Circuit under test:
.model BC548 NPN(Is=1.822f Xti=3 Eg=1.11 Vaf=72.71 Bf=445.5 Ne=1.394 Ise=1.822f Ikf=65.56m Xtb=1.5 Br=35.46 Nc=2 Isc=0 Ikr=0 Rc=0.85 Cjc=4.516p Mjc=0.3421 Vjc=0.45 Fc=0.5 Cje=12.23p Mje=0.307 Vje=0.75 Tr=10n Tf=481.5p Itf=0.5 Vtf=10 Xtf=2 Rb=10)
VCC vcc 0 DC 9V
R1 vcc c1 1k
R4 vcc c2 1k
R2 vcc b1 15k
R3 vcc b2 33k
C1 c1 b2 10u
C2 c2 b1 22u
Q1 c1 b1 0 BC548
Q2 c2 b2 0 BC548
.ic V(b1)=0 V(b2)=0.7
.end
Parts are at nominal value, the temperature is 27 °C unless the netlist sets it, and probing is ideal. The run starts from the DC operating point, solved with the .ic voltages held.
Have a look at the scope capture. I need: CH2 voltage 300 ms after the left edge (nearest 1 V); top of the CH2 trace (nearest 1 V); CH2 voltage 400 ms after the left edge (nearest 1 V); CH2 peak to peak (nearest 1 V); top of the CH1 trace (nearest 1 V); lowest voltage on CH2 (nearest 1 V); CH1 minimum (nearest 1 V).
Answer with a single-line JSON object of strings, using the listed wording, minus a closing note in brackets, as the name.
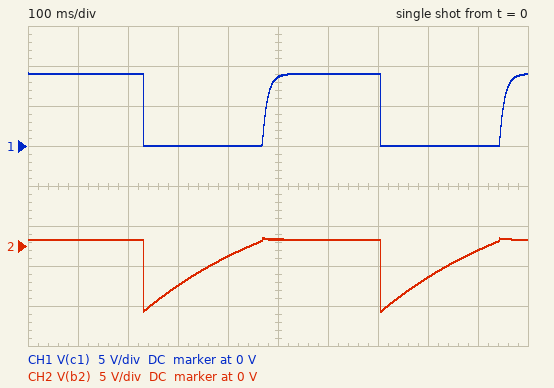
{"CH2 voltage 300 ms after the left edge": "-5 V", "top of the CH2 trace": "1 V", "CH2 voltage 400 ms after the left edge": "-1 V", "CH2 peak to peak": "9 V", "top of the CH1 trace": "9 V", "lowest voltage on CH2": "-8 V", "CH1 minimum": "0 V"}
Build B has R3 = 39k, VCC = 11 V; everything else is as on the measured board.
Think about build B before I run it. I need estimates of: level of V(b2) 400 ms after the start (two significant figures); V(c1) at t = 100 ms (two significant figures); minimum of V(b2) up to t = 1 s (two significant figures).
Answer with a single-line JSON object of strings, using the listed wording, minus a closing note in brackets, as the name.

{"level of V(b2) 400 ms after the start": "-2.7 V", "V(c1) at t = 100 ms": "11 V", "minimum of V(b2) up to t = 1 s": "-10 V"}
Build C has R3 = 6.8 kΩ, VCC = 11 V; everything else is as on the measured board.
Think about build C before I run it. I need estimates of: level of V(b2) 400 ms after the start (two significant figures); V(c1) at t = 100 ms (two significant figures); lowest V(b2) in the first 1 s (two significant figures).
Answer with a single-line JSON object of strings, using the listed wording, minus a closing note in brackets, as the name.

{"level of V(b2) 400 ms after the start": "820 mV", "V(c1) at t = 100 ms": "11 V", "lowest V(b2) in the first 1 s": "-10 V"}
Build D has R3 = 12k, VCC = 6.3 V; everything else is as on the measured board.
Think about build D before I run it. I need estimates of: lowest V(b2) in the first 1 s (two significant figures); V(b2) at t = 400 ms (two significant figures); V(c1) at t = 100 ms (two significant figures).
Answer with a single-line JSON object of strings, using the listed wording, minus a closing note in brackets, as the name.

{"lowest V(b2) in the first 1 s": "-5.5 V", "V(b2) at t = 400 ms": "790 mV", "V(c1) at t = 100 ms": "6.3 V"}
